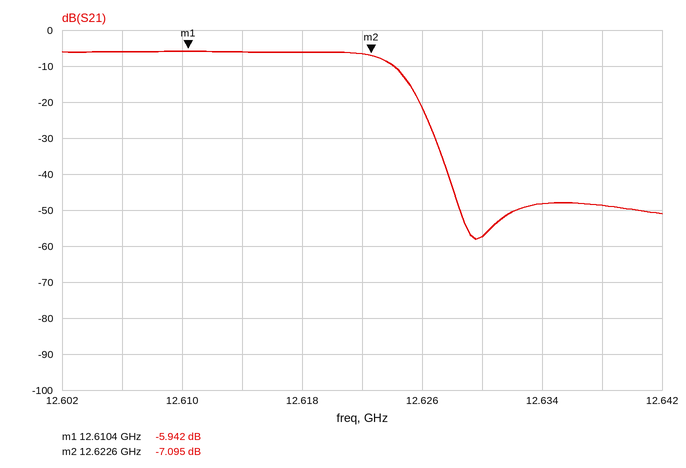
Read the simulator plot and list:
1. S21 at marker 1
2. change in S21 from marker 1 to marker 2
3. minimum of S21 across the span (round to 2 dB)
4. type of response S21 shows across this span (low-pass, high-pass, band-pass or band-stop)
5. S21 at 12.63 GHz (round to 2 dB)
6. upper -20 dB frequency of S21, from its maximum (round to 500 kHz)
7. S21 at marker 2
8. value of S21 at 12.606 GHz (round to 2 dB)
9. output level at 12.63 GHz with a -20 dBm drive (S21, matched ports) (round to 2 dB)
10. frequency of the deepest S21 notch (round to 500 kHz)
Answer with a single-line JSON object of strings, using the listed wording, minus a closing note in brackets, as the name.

{"S21 at marker 1": "-5.942 dB", "change in S21 from marker 1 to marker 2": "-1.153 dB", "minimum of S21 across the span": "-58 dB", "type of response S21 shows across this span": "low-pass", "S21 at 12.63 GHz": "-58 dB", "upper -20 dB frequency of S21, from its maximum": "12.6265 GHz", "S21 at marker 2": "-7.095 dB", "value of S21 at 12.606 GHz": "-6 dB", "output level at 12.63 GHz with a -20 dBm drive (S21, matched ports)": "-78 dBm", "frequency of the deepest S21 notch": "12.6295 GHz"}
